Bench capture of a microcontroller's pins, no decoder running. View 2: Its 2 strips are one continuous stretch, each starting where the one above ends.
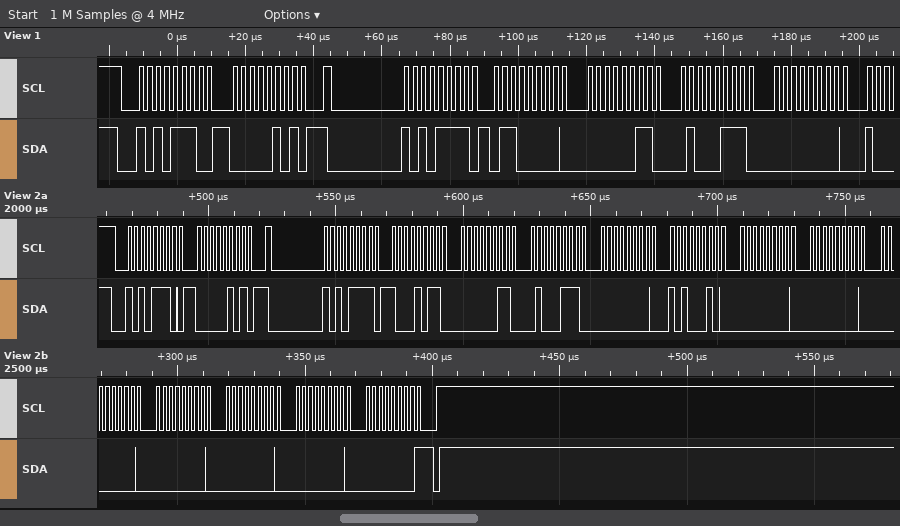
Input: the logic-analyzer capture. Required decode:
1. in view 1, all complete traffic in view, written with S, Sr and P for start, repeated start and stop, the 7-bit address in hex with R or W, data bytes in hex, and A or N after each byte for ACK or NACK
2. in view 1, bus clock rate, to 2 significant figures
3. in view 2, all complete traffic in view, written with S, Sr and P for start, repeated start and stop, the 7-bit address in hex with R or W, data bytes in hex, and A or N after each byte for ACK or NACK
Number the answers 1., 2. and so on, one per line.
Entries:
1. S 57W A 05 A Sr 57R A 60 A 03 A 47 A 00 A
2. 400 kHz
3. S 57W A 05 A Sr 57R A 8B A 03 A 47 A 00 A A2 A 00 A 00 A 00 A 00 A 00 A 00 A 00 N P
